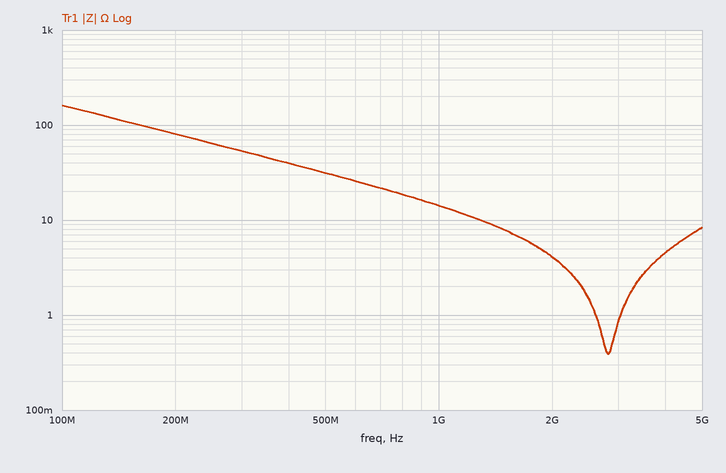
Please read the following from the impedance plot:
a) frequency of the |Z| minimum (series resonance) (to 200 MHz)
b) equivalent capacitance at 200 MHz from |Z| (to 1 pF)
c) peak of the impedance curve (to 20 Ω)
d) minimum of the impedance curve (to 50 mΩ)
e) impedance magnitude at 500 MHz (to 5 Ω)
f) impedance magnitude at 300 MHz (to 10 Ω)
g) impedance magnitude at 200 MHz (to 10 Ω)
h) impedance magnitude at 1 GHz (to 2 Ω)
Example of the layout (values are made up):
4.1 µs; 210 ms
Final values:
2.8 GHz; 10 pF; 160 Ω; 400 mΩ; 30 Ω; 50 Ω; 80 Ω; 14 Ω
